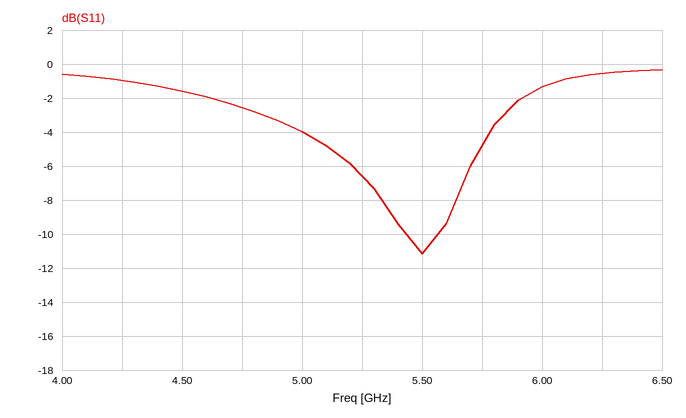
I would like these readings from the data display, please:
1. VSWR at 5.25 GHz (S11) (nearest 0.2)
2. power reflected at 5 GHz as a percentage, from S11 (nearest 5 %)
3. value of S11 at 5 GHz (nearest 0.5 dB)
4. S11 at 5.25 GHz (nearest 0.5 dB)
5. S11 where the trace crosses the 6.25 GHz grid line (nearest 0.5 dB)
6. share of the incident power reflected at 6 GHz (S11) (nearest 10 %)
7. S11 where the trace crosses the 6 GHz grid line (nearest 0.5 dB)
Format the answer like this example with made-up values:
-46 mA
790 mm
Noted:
2.8
40 %
-4.0 dB
-6.5 dB
-0.5 dB
70 %
-1.5 dB
